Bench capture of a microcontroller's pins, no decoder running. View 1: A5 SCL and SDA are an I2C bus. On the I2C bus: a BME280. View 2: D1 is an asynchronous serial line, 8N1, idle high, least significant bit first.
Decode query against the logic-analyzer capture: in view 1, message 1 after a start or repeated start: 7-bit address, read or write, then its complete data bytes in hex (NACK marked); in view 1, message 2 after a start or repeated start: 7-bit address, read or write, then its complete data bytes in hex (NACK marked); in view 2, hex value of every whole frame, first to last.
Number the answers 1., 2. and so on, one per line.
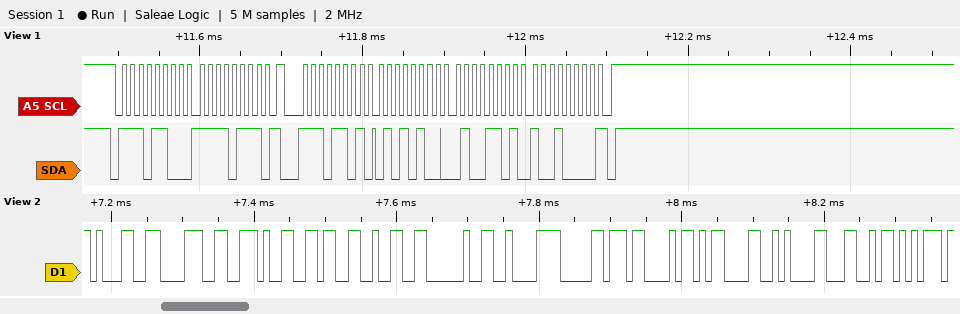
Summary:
1. 0x76 write: F7
2. 0x76 read: 54 4D 90 NACK
3. 31 38 2E 36 32 20 C2 B0 43 0D 0A 4C 75
